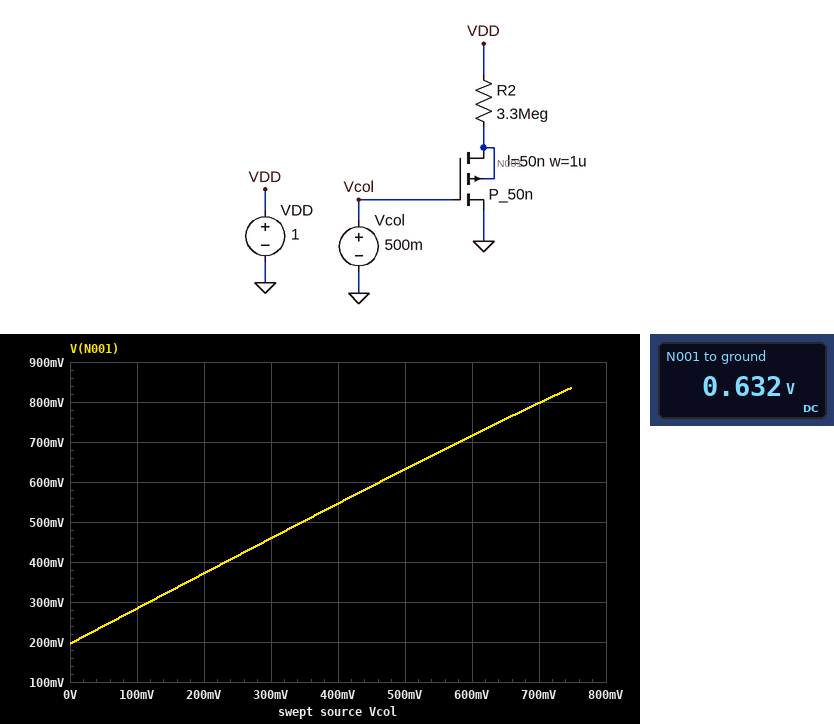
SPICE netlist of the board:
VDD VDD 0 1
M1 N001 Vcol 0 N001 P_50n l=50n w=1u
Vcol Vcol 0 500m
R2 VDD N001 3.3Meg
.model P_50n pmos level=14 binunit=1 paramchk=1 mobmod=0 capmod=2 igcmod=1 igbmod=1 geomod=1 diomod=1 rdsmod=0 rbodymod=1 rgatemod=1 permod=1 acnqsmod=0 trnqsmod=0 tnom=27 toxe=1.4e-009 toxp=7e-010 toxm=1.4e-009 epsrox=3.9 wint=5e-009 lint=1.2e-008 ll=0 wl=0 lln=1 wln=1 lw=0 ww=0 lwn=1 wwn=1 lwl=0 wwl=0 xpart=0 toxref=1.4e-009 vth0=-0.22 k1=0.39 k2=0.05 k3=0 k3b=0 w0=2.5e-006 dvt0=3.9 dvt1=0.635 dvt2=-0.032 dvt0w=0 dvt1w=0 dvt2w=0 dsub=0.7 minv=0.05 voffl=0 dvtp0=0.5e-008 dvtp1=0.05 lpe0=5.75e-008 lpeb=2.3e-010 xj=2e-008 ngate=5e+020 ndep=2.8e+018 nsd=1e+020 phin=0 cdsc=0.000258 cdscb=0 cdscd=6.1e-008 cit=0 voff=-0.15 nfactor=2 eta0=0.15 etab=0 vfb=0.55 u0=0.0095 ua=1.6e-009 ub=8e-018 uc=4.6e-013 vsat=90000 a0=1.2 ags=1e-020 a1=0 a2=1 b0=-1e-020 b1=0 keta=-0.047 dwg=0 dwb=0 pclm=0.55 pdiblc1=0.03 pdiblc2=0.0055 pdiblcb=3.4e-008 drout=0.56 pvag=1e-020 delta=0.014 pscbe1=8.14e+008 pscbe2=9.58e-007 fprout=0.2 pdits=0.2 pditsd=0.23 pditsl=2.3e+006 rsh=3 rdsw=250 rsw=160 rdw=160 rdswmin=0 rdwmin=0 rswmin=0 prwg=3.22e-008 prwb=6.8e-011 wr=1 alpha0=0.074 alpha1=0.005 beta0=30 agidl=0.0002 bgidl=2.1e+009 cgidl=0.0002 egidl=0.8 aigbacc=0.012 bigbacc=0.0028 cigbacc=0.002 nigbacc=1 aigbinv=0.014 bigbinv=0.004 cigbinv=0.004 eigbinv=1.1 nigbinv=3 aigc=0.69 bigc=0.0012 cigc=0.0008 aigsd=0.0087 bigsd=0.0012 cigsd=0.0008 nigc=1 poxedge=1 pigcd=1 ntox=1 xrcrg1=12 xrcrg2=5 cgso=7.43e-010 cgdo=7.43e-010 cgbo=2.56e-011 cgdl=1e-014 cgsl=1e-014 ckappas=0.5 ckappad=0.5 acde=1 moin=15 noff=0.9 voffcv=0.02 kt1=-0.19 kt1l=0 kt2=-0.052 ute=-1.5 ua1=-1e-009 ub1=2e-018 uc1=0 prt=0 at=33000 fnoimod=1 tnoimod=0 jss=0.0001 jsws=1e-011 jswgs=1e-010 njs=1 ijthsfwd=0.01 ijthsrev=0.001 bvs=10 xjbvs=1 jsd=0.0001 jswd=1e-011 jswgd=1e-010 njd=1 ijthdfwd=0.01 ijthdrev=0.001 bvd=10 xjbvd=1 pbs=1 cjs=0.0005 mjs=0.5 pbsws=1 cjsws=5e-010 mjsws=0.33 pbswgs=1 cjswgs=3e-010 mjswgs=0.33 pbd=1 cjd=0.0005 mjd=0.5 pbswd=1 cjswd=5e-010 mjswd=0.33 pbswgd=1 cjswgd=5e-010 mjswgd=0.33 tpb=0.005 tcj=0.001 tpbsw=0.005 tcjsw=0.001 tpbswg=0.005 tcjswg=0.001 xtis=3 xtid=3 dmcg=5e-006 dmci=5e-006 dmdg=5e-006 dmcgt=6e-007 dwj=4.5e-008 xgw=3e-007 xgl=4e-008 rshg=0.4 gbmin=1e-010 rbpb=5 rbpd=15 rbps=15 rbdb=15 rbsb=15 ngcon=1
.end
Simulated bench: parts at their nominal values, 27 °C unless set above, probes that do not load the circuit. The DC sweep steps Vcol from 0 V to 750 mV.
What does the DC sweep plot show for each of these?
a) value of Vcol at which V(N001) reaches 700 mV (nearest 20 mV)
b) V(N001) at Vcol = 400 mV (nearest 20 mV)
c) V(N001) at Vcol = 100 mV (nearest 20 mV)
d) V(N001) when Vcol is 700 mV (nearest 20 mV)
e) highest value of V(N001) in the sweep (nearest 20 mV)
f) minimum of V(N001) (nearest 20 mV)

580 mV
540 mV
280 mV
800 mV
840 mV
200 mV
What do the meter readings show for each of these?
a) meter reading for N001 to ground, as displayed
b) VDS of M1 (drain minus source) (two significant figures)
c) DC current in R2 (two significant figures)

0.632 V
630 mV
110 nA
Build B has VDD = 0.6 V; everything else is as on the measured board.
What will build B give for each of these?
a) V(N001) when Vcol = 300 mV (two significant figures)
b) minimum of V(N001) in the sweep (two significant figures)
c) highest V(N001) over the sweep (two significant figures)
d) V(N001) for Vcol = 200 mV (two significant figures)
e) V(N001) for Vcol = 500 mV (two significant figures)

420 mV
170 mV
600 mV
340 mV
550 mV
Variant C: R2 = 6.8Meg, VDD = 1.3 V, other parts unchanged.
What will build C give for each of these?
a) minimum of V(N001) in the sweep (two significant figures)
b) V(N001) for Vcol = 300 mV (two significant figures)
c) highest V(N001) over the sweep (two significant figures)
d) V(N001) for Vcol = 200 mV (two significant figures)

180 mV
450 mV
850 mV
360 mV
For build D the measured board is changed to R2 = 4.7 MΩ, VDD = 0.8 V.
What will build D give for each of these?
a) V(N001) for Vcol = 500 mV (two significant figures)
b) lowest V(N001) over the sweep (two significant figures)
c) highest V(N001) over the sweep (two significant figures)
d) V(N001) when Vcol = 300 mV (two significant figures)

600 mV
170 mV
770 mV
430 mV
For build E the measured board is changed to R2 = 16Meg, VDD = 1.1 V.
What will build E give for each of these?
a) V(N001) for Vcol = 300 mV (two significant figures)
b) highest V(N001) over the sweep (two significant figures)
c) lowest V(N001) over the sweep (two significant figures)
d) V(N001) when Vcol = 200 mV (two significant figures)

410 mV
800 mV
140 mV
320 mV
